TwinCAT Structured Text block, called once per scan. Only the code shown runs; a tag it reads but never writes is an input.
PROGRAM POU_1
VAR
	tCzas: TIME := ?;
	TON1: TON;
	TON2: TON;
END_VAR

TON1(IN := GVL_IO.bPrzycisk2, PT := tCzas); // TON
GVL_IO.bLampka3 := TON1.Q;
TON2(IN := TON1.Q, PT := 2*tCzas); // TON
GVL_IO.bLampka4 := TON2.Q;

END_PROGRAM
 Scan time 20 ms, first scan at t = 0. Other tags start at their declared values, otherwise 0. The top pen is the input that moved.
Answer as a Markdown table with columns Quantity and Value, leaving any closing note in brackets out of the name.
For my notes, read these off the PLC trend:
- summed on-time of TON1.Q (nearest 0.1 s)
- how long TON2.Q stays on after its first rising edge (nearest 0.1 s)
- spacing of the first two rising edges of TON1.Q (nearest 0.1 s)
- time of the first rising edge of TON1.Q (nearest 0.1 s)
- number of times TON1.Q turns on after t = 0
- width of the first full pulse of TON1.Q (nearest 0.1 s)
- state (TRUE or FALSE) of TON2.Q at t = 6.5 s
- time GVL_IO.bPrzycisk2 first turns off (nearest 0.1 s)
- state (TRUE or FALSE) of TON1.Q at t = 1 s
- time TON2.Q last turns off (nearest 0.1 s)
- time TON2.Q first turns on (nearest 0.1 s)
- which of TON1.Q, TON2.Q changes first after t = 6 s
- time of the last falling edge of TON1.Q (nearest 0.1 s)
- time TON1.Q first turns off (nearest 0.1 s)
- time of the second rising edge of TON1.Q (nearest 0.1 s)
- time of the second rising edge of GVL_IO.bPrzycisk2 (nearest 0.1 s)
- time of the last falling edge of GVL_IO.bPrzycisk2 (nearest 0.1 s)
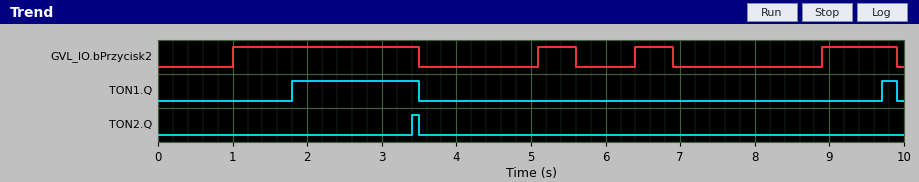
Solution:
| Quantity | Value |
|---|---|
| summed on-time of TON1.Q | 1.9 s |
| how long TON2.Q stays on after its first rising edge | 0.1 s |
| spacing of the first two rising edges of TON1.Q | 7.9 s |
| time of the first rising edge of TON1.Q | 1.8 s |
| number of times TON1.Q turns on after t = 0 | 2 |
| width of the first full pulse of TON1.Q | 1.7 s |
| state (TRUE or FALSE) of TON2.Q at t = 6.5 s | FALSE |
| time GVL_IO.bPrzycisk2 first turns off | 3.5 s |
| state (TRUE or FALSE) of TON1.Q at t = 1 s | FALSE |
| time TON2.Q last turns off | 3.5 s |
| time TON2.Q first turns on | 3.4 s |
| which of TON1.Q, TON2.Q changes first after t = 6 s | TON1.Q |
| time of the last falling edge of TON1.Q | 9.9 s |
| time TON1.Q first turns off | 3.5 s |
| time of the second rising edge of TON1.Q | 9.7 s |
| time of the second rising edge of GVL_IO.bPrzycisk2 | 5.1 s |
| time of the last falling edge of GVL_IO.bPrzycisk2 | 9.9 s |
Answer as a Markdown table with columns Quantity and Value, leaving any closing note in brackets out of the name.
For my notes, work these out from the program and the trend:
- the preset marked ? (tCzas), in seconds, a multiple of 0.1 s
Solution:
| Quantity | Value |
|---|---|
| the preset marked ? (tCzas), in seconds, a multiple of 0.1 s | 0.8 s |
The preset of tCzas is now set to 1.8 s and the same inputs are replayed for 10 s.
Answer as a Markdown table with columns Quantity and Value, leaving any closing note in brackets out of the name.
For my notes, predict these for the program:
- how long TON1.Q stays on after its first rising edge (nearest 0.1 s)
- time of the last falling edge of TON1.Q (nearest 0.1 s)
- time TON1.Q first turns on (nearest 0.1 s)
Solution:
| Quantity | Value |
|---|---|
| how long TON1.Q stays on after its first rising edge | 0.7 s |
| time of the last falling edge of TON1.Q | 3.5 s |
| time TON1.Q first turns on | 2.8 s |
